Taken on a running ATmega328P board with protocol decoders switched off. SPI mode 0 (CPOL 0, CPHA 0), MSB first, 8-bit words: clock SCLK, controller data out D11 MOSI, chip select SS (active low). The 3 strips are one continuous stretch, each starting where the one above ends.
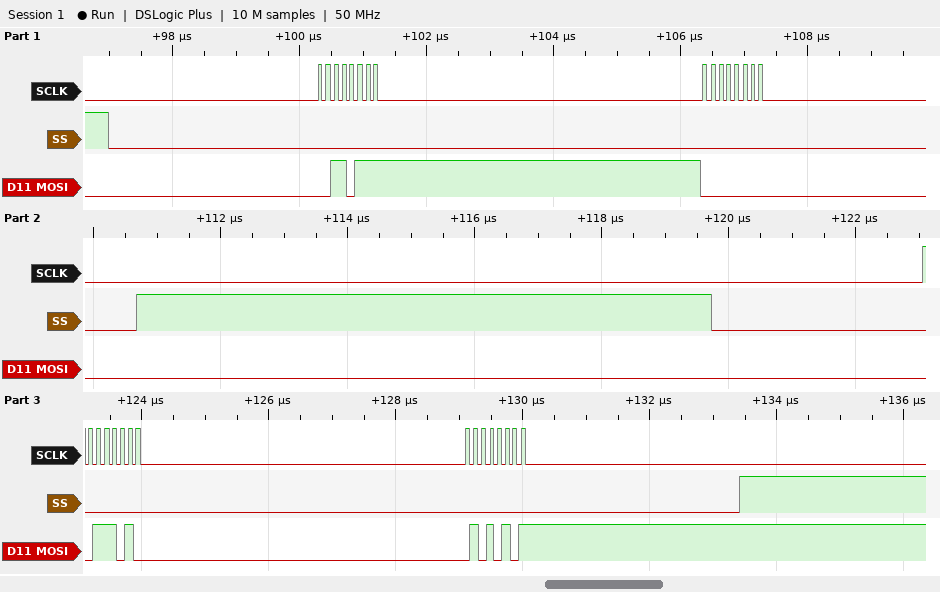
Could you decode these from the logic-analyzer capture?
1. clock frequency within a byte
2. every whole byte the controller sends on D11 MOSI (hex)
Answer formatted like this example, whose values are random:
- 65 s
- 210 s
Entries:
- 8 MHz
- 37 00 3A 55
